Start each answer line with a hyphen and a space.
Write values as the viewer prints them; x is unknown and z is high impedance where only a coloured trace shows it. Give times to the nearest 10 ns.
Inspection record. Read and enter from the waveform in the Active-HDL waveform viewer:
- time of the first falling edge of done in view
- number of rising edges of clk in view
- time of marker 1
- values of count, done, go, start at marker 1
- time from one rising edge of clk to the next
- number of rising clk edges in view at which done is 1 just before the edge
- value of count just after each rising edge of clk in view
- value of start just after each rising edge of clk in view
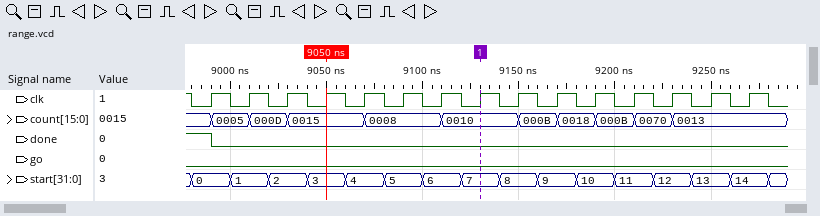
- 8990 ns
- 15
- 9130 ns
- count=0010, done=0, go=0, start=7
- 20 ns
- 1
- 0005, 000D, 0015, 0015, 0008, 0008, 0010, 0010, 000B, 0018, 000B, 0070, 0013, 0013, 0013
- 0, 1, 2, 3, 4, 5, 6, 7, 8, 9, 10, 11, 12, 13, 14
